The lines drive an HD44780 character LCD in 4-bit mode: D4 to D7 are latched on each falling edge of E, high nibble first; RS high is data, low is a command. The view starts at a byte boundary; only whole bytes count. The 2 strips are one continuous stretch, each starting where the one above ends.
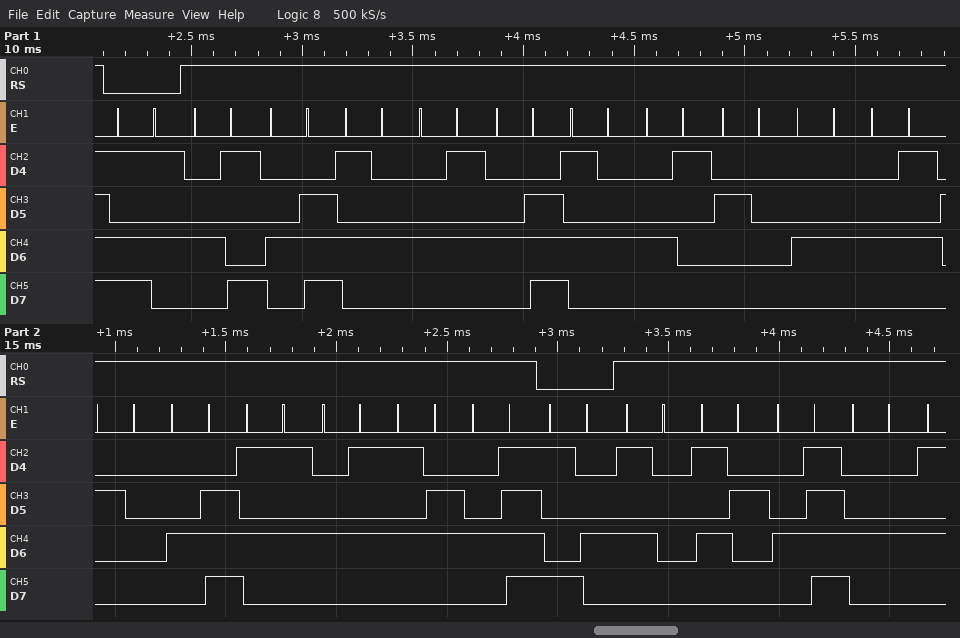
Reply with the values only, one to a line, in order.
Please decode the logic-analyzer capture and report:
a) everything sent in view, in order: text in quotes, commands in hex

0xD5 "INTENTA DE NUEVO" 0x94 "PROD"
